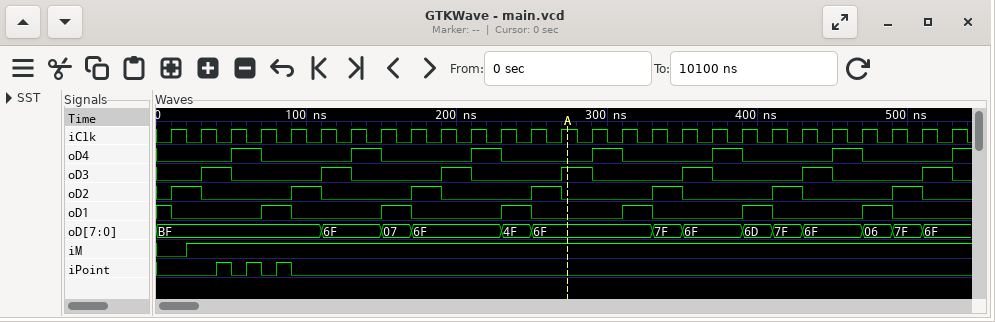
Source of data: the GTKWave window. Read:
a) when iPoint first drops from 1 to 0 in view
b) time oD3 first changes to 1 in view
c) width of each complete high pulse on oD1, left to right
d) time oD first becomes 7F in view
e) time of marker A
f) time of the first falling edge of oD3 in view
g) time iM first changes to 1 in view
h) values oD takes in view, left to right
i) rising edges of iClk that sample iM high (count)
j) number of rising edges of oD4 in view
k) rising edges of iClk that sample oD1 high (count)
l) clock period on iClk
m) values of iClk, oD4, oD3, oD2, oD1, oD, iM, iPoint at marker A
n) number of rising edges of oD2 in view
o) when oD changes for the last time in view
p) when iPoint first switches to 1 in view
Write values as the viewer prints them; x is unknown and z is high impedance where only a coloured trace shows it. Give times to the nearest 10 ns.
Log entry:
50 ns
30 ns
20 ns, 20 ns, 20 ns, 20 ns, 20 ns, 20 ns
330 ns
270 ns
50 ns
20 ns
BF, 6F, 07, 6F, 4F, 6F, 7F, 6F, 6D, 7F, 6F, 06, 7F, 6F
26
7
7
20 ns
iClk=1, oD4=0, oD3=1, oD2=0, oD1=0, oD=6F, iM=1, iPoint=0
7
510 ns
40 ns
